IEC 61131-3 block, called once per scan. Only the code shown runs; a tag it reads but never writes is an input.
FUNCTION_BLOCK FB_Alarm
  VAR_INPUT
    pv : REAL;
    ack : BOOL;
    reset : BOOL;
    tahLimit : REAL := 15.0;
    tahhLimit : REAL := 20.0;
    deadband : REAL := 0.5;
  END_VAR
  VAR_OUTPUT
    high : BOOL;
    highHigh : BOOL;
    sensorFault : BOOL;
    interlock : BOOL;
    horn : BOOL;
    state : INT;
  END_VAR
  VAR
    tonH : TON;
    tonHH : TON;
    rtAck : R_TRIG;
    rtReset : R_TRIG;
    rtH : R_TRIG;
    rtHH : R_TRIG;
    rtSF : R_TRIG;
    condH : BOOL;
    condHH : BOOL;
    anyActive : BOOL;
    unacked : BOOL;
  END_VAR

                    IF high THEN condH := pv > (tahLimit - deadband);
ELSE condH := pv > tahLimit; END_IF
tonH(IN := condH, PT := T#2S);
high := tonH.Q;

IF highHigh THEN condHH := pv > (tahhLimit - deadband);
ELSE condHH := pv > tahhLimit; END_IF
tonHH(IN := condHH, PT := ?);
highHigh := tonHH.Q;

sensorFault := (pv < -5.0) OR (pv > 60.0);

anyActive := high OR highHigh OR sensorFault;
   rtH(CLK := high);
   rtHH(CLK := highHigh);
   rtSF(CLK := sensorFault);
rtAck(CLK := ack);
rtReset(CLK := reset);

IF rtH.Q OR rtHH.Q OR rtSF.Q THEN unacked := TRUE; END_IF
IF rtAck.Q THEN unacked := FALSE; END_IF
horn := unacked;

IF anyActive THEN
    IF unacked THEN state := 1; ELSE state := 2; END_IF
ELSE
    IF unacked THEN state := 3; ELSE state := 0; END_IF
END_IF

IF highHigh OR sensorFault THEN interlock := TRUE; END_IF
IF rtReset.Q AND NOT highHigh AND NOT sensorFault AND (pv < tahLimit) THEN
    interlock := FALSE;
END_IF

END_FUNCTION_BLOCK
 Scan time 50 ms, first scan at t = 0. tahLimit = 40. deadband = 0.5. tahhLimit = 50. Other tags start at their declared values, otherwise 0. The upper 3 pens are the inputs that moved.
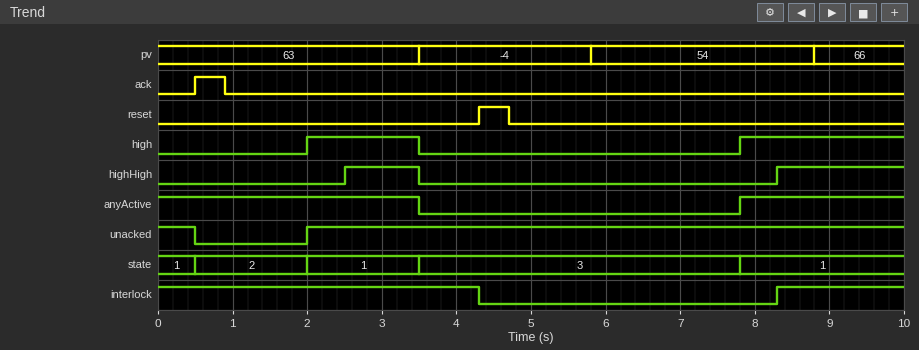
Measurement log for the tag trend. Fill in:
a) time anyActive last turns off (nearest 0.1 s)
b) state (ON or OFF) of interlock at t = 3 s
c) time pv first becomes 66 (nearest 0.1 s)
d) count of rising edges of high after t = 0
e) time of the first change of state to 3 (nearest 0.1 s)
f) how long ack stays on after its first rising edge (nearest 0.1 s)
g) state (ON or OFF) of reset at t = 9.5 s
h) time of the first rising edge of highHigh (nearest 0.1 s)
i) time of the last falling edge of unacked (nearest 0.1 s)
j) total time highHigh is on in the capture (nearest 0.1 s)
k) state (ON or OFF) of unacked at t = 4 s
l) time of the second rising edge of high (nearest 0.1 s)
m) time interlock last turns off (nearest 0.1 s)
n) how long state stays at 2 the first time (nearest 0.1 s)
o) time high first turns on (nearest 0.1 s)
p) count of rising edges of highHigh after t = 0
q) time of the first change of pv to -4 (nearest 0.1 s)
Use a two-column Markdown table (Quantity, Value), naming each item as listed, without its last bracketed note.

| Quantity | Value |
|---|---|
| time anyActive last turns off | 3.5 s |
| state (ON or OFF) of interlock at t = 3 s | ON |
| time pv first becomes 66 | 8.8 s |
| count of rising edges of high after t = 0 | 2 |
| time of the first change of state to 3 | 3.5 s |
| how long ack stays on after its first rising edge | 0.4 s |
| state (ON or OFF) of reset at t = 9.5 s | OFF |
| time of the first rising edge of highHigh | 2.5 s |
| time of the last falling edge of unacked | 0.5 s |
| total time highHigh is on in the capture | 2.7 s |
| state (ON or OFF) of unacked at t = 4 s | ON |
| time of the second rising edge of high | 7.8 s |
| time interlock last turns off | 4.3 s |
| how long state stays at 2 the first time | 1.5 s |
| time high first turns on | 2.0 s |
| count of rising edges of highHigh after t = 0 | 2 |
| time of the first change of pv to -4 | 3.5 s |
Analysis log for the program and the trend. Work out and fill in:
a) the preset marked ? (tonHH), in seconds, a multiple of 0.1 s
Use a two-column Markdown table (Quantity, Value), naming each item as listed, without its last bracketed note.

| Quantity | Value |
|---|---|
| the preset marked ? (tonHH), in seconds, a multiple of 0.1 s | 2.5 s |
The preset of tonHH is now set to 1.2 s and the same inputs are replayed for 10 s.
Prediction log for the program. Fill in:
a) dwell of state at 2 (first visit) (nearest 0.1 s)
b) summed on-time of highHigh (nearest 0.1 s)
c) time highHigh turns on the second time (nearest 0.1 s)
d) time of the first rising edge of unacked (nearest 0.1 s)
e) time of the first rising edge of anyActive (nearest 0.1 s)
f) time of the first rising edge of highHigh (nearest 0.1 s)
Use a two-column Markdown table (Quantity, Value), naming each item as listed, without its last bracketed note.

| Quantity | Value |
|---|---|
| dwell of state at 2 (first visit) | 0.7 s |
| summed on-time of highHigh | 5.3 s |
| time highHigh turns on the second time | 7.0 s |
| time of the first rising edge of unacked | 1.2 s |
| time of the first rising edge of anyActive | 7.0 s |
| time of the first rising edge of highHigh | 1.2 s |
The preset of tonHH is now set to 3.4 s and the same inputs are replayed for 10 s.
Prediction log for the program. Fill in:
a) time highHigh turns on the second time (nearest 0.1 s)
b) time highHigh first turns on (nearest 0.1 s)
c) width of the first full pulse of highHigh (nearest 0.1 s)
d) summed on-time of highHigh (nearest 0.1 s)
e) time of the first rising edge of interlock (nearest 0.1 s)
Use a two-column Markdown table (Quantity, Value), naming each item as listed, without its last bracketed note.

| Quantity | Value |
|---|---|
| time highHigh turns on the second time | 9.2 s |
| time highHigh first turns on | 3.4 s |
| width of the first full pulse of highHigh | 0.1 s |
| summed on-time of highHigh | 0.9 s |
| time of the first rising edge of interlock | 8.8 s |
